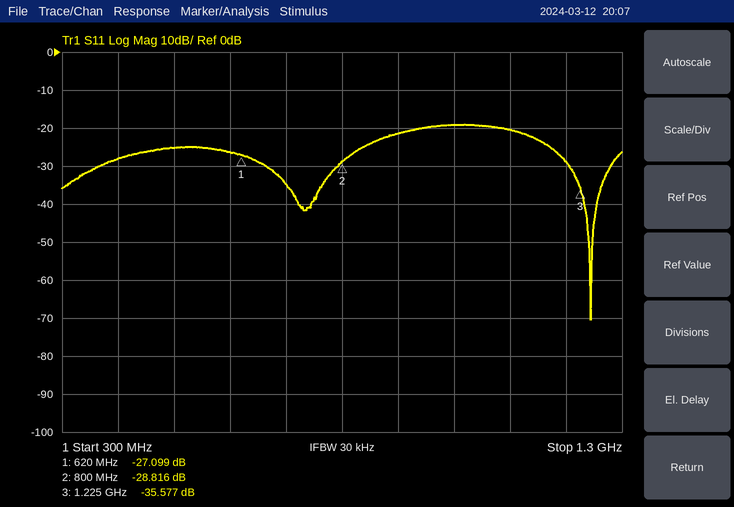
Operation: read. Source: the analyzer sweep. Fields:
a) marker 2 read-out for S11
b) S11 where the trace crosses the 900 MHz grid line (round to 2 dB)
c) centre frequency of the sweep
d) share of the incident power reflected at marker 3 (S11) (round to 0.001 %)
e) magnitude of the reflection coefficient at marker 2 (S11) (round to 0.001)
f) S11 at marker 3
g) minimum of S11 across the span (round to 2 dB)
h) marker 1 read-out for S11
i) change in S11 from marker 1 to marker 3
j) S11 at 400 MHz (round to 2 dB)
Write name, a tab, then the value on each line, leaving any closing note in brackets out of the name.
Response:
marker 2 read-out for S11	-28.816 dB
S11 where the trace crosses the 900 MHz grid line	-22 dB
centre frequency of the sweep	800 MHz
share of the incident power reflected at marker 3 (S11)	0.028 %
magnitude of the reflection coefficient at marker 2 (S11)	0.036
S11 at marker 3	-35.577 dB
minimum of S11 across the span	-70 dB
marker 1 read-out for S11	-27.099 dB
change in S11 from marker 1 to marker 3	-8.478 dB
S11 at 400 MHz	-28 dB
